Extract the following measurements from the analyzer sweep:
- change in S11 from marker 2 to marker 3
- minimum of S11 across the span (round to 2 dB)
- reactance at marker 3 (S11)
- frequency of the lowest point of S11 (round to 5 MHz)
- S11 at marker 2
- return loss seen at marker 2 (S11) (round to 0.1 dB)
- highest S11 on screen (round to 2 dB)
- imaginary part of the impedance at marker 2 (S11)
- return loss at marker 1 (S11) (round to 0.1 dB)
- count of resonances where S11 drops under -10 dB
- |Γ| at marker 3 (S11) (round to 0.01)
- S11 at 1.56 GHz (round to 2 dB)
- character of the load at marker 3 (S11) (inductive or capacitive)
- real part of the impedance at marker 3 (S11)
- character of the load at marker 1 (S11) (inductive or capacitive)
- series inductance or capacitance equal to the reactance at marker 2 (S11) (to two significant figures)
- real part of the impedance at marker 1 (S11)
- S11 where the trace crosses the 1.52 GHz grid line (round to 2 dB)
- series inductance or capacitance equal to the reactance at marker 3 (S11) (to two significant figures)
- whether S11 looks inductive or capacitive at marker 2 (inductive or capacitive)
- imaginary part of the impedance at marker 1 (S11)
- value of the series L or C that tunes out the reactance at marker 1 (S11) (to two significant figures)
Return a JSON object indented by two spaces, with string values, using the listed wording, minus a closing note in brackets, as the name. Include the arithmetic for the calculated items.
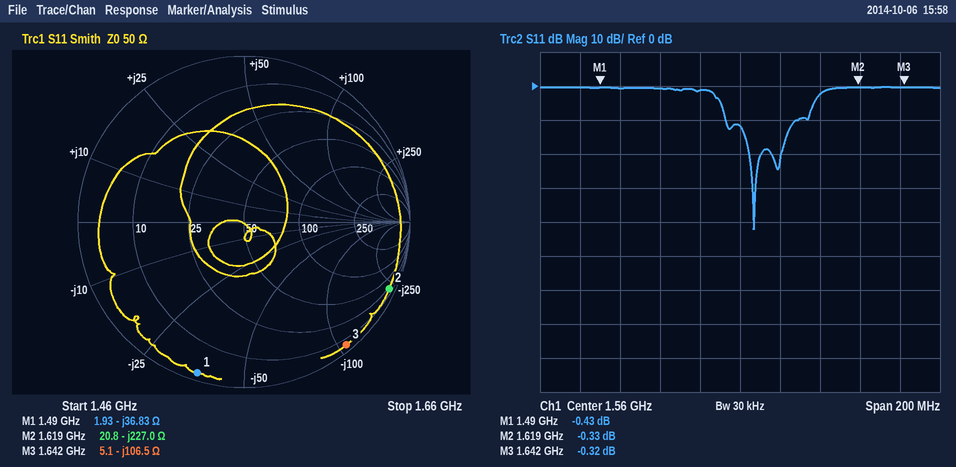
{
  "change in S11 from marker 2 to marker 3": "-0.32 − (-0.33) = 0.01 dB",
  "minimum of S11 across the span": "-42 dB",
  "reactance at marker 3": "-106.5 Ω",
  "frequency of the lowest point of S11": "1.565 GHz",
  "S11 at marker 2": "-0.33 dB",
  "return loss seen at marker 2 (S11)": "0.3 dB",
  "highest S11 on screen": "0 dB",
  "imaginary part of the impedance at marker 2": "-227.0 Ω",
  "return loss at marker 1 (S11)": "0.4 dB",
  "count of resonances where S11 drops under -10 dB": "2",
  "|Γ| at marker 3 (S11)": "0.96",
  "S11 at 1.56 GHz": "-12 dB",
  "character of the load at marker 3 (S11)": "capacitive",
  "real part of the impedance at marker 3": "5.1 Ω",
  "character of the load at marker 1 (S11)": "capacitive",
  "series inductance or capacitance equal to the reactance at marker 2 (S11)": "C = 1/(2π × 1.619 GHz × 227 Ω) ≈ 433 fF, so 430 fF to two significant figures",
  "real part of the impedance at marker 1": "1.93 Ω",
  "S11 where the trace crosses the 1.52 GHz grid line": "0 dB",
  "series inductance or capacitance equal to the reactance at marker 3 (S11)": "C = 1/(2π × 1.642 GHz × 106.5 Ω) ≈ 910 fF",
  "whether S11 looks inductive or capacitive at marker 2": "capacitive",
  "imaginary part of the impedance at marker 1": "-36.83 Ω",
  "value of the series L or C that tunes out the reactance at marker 1 (S11)": "L = 36.83 Ω/(2π × 1.49 GHz) ≈ 3.9 nH"
}
